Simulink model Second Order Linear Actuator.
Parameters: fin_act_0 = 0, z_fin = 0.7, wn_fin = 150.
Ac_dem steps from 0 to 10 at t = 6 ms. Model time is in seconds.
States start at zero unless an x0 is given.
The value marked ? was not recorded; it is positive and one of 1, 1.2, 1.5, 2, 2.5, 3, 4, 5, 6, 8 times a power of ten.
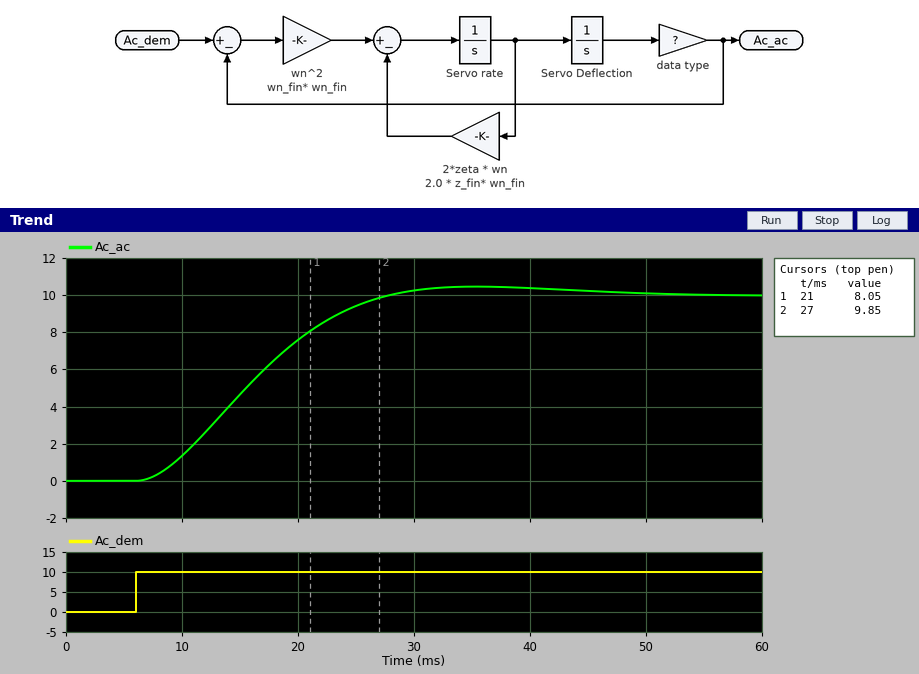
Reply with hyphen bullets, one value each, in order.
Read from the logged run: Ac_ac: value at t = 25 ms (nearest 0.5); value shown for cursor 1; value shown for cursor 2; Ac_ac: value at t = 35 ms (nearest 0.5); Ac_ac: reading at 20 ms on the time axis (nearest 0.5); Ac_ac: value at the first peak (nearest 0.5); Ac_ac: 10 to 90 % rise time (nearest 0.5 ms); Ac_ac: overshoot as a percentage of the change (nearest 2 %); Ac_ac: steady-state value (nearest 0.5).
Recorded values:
- 9.5
- 8.05
- 9.85
- 10.5
- 7.5
- 10.5
- 14.0 ms
- 4 %
- 10.0
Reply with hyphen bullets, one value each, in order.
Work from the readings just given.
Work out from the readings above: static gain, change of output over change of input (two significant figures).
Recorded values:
- 1.0
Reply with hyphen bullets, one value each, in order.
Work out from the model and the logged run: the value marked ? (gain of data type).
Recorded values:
- 1
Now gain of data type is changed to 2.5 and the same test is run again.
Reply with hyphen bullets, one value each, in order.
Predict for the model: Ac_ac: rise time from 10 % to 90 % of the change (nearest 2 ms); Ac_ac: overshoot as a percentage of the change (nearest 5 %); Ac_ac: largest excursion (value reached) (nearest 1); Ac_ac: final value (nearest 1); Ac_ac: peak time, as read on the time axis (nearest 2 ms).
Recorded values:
- 6 ms
- 20 %
- 12
- 10
- 20 ms
